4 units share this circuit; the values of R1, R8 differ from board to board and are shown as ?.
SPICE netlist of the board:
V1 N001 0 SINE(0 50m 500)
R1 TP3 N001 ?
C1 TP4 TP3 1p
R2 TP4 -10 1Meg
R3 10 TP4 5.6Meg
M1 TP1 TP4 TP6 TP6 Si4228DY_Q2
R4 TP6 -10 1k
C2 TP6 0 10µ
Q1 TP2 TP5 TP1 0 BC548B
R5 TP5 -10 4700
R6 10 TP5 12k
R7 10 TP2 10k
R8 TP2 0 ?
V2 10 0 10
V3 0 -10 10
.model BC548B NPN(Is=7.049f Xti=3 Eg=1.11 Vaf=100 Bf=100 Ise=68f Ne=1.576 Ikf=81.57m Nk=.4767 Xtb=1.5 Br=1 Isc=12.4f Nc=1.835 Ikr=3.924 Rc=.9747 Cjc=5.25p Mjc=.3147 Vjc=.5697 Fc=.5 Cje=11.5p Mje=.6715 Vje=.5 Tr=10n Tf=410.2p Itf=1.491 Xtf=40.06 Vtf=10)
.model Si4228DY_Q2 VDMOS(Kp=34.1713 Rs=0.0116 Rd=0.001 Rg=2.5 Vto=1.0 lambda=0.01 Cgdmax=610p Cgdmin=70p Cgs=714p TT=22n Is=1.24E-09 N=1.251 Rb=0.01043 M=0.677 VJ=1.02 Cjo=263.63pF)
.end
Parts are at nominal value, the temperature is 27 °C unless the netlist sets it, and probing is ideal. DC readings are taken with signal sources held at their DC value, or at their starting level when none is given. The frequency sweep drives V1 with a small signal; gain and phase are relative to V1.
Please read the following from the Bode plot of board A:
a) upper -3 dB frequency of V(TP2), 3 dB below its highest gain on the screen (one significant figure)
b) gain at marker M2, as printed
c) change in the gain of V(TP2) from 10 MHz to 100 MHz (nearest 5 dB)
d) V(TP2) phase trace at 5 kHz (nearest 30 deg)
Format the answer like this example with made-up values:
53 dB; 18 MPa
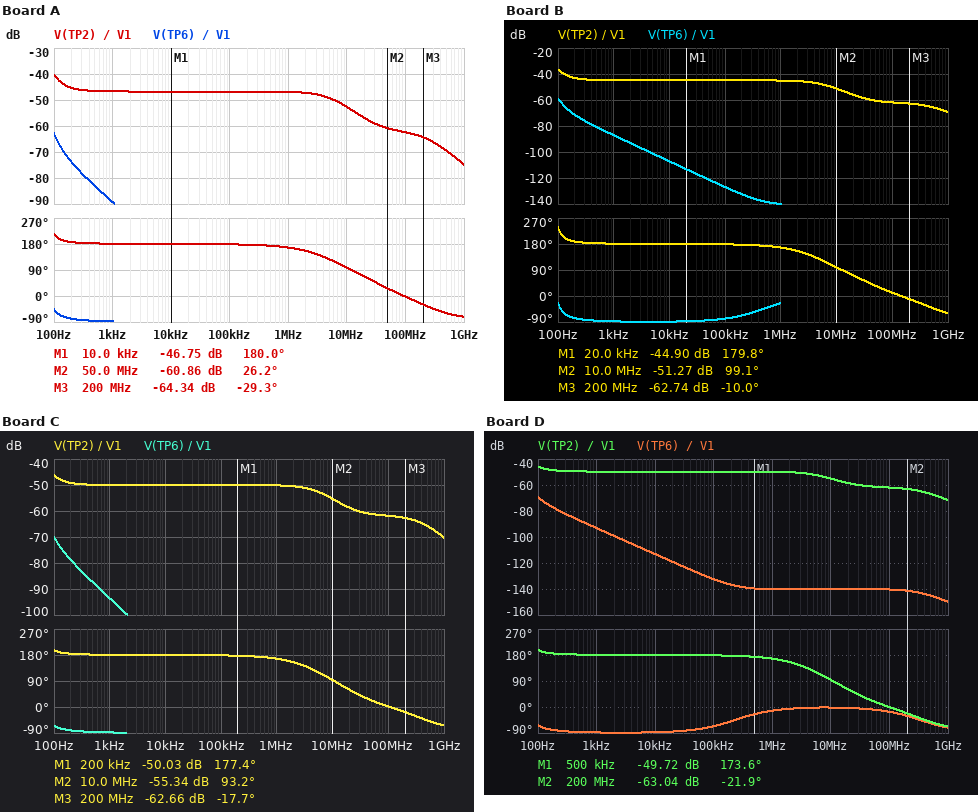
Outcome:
100 Hz; -60.86 dB; -10 dB; 180 deg
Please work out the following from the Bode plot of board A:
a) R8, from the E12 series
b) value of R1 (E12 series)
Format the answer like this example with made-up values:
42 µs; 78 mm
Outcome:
12 kΩ; 680 Ω
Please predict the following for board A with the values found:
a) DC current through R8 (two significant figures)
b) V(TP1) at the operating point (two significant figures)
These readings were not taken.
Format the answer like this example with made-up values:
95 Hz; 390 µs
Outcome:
470 µA; -5.7 V
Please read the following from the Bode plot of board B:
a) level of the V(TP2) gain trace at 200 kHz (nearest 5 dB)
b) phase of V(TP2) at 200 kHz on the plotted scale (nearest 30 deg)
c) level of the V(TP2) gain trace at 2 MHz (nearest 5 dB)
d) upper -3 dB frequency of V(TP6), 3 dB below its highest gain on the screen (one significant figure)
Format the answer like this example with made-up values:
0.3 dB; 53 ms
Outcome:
-45 dB; 180 deg; -45 dB; 100 Hz
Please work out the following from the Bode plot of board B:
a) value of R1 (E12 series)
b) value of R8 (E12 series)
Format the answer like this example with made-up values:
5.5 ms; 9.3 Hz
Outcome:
330 Ω; 8.2 kΩ
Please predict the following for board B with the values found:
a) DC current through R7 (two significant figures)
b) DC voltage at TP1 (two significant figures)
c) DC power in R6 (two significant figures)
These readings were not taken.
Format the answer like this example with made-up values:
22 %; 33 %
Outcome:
1.5 mA; -5.3 V; 18 mW
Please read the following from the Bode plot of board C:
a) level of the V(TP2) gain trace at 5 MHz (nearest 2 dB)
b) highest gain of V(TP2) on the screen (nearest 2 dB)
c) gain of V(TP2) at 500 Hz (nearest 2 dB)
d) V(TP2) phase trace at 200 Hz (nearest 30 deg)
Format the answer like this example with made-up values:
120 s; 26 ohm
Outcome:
-52 dB; -46 dB; -50 dB; 180 deg
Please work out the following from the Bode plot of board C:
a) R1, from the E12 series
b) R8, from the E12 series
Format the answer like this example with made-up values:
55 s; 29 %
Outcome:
390 Ω; 39 kΩ
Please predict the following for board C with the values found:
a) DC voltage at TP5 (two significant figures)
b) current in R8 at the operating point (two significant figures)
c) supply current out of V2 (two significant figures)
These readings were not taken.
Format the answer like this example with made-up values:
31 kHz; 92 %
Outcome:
-5.8 V; 170 µA; 3.0 mA
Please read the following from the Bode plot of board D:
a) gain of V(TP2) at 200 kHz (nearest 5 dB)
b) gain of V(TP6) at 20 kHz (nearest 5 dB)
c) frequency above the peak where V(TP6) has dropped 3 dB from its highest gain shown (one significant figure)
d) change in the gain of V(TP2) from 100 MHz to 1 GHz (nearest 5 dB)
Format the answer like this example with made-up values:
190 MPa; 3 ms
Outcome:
-50 dB; -120 dB; 100 Hz; -10 dB
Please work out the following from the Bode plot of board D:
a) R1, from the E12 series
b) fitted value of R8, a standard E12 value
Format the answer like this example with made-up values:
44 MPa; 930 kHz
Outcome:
470 Ω; 33 kΩ
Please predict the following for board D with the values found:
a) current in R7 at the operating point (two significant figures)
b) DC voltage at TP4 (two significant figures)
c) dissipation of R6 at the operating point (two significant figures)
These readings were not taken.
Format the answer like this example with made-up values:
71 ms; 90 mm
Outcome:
1.6 mA; -7.0 V; 21 mW
